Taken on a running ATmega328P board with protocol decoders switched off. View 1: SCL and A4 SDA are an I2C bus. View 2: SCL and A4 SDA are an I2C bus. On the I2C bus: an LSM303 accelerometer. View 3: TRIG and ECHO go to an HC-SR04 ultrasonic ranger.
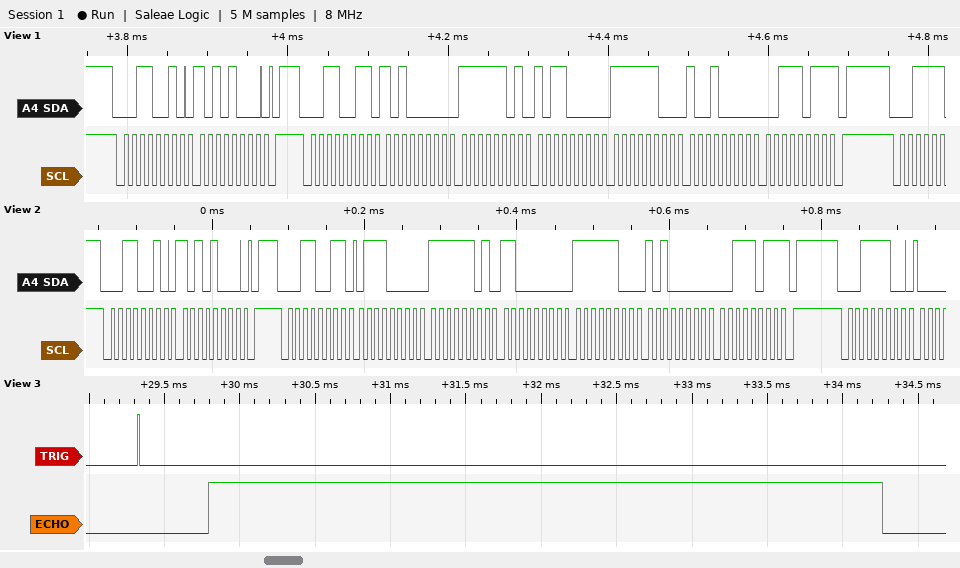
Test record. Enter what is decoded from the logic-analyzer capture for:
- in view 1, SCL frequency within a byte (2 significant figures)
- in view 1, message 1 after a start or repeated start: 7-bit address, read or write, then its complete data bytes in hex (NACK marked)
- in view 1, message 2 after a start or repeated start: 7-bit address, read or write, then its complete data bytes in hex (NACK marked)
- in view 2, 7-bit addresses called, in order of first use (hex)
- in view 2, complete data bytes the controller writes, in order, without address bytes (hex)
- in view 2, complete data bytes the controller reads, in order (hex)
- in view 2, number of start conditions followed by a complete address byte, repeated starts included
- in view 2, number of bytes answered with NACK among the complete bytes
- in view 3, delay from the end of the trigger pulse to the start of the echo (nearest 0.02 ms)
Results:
100 kHz
0x19 write: A8
0x19 read: A0 FD B0 FC 90 3B NACK
0x19 0x1E
A8
70 FD C0 FC A0 3B
3
1
0.46 ms
